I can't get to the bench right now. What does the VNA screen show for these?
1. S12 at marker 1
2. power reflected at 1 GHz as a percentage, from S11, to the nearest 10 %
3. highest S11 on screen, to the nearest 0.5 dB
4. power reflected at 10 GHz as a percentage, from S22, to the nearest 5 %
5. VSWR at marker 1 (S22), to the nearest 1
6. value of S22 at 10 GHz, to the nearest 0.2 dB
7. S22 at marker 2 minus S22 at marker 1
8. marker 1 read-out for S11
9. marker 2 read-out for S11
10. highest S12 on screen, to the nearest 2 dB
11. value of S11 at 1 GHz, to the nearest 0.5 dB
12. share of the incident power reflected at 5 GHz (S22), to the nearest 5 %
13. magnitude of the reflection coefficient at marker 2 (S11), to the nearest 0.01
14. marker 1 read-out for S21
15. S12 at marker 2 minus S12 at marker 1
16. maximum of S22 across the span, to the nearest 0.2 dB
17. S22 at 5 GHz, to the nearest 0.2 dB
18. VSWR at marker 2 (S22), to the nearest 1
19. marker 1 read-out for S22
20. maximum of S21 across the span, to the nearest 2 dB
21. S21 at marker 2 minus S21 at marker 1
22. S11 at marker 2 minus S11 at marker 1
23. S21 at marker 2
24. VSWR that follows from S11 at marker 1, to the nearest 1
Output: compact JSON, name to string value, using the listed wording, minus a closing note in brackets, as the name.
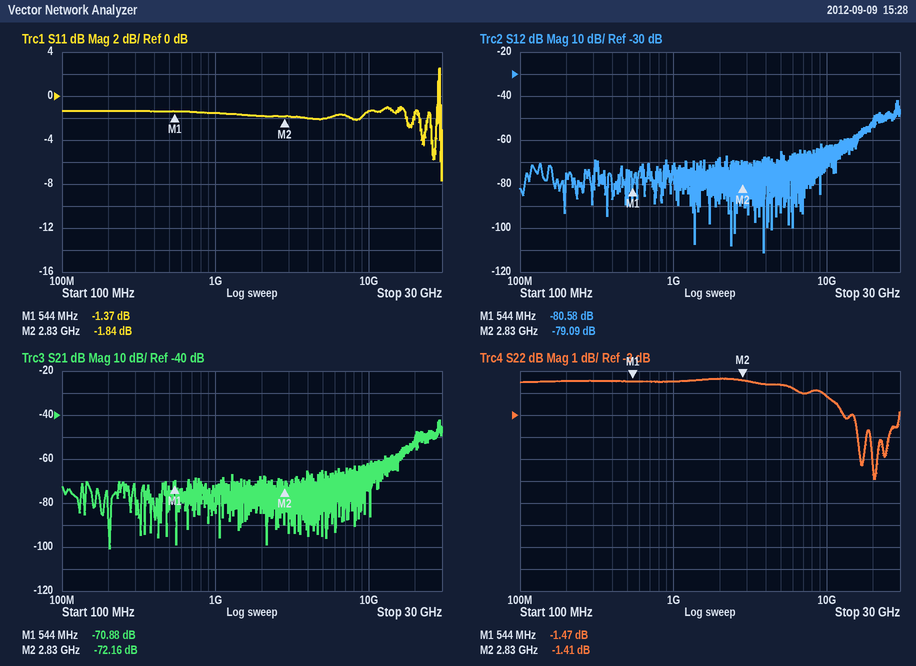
{"S12 at marker 1": "-80.58 dB", "power reflected at 1 GHz as a percentage, from S11, to the nearest 10 %": "70 %", "highest S11 on screen, to the nearest 0.5 dB": "2.5 dB", "power reflected at 10 GHz as a percentage, from S22, to the nearest 5 %": "60 %", "VSWR at marker 1 (S22), to the nearest 1": "12", "value of S22 at 10 GHz, to the nearest 0.2 dB": "-2.2 dB", "S22 at marker 2 minus S22 at marker 1": "0.06 dB", "marker 1 read-out for S11": "-1.37 dB", "marker 2 read-out for S11": "-1.84 dB", "highest S12 on screen, to the nearest 2 dB": "-42 dB", "value of S11 at 1 GHz, to the nearest 0.5 dB": "-1.5 dB", "share of the incident power reflected at 5 GHz (S22), to the nearest 5 %": "70 %", "magnitude of the reflection coefficient at marker 2 (S11), to the nearest 0.01": "0.81", "marker 1 read-out for S21": "-70.88 dB", "S12 at marker 2 minus S12 at marker 1": "1.49 dB", "maximum of S22 across the span, to the nearest 0.2 dB": "-1.4 dB", "S22 at 5 GHz, to the nearest 0.2 dB": "-1.6 dB", "VSWR at marker 2 (S22), to the nearest 1": "12", "marker 1 read-out for S22": "-1.47 dB", "maximum of S21 across the span, to the nearest 2 dB": "-42 dB", "S21 at marker 2 minus S21 at marker 1": "-1.28 dB", "S11 at marker 2 minus S11 at marker 1": "-0.47 dB", "S21 at marker 2": "-72.16 dB", "VSWR that follows from S11 at marker 1, to the nearest 1": "13"}
